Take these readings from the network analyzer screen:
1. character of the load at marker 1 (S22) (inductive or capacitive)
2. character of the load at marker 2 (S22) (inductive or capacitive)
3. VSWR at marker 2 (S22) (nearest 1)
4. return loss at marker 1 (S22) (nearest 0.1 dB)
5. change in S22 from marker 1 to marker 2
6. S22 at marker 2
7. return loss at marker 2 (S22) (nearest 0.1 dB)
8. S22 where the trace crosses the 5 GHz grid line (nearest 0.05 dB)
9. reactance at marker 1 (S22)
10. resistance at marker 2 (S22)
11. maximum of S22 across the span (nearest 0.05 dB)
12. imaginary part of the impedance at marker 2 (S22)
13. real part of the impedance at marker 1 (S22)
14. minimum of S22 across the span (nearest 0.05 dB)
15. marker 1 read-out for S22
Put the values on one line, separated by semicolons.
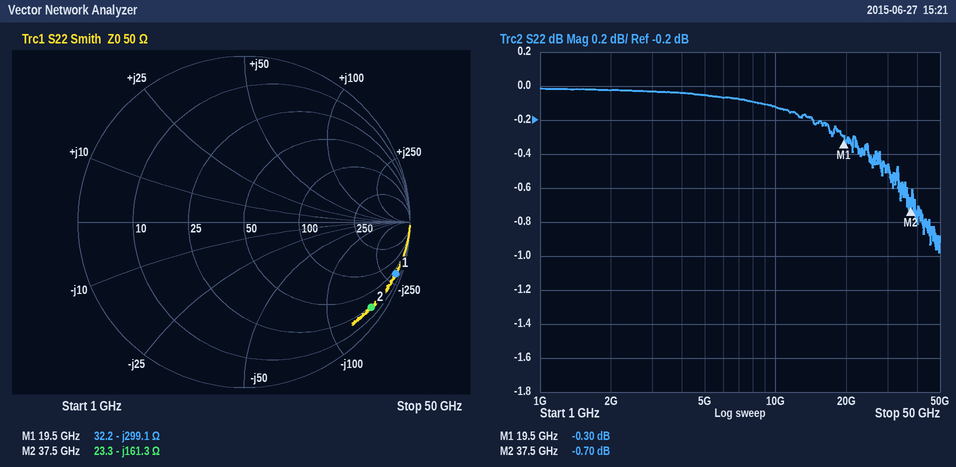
capacitive; capacitive; 25; 0.3 dB; -0.40 dB; -0.70 dB; 0.7 dB; -0.05 dB; -299.1 Ω; 23.3 Ω; 0.00 dB; -161.3 Ω; 32.2 Ω; -1.00 dB; -0.30 dB
